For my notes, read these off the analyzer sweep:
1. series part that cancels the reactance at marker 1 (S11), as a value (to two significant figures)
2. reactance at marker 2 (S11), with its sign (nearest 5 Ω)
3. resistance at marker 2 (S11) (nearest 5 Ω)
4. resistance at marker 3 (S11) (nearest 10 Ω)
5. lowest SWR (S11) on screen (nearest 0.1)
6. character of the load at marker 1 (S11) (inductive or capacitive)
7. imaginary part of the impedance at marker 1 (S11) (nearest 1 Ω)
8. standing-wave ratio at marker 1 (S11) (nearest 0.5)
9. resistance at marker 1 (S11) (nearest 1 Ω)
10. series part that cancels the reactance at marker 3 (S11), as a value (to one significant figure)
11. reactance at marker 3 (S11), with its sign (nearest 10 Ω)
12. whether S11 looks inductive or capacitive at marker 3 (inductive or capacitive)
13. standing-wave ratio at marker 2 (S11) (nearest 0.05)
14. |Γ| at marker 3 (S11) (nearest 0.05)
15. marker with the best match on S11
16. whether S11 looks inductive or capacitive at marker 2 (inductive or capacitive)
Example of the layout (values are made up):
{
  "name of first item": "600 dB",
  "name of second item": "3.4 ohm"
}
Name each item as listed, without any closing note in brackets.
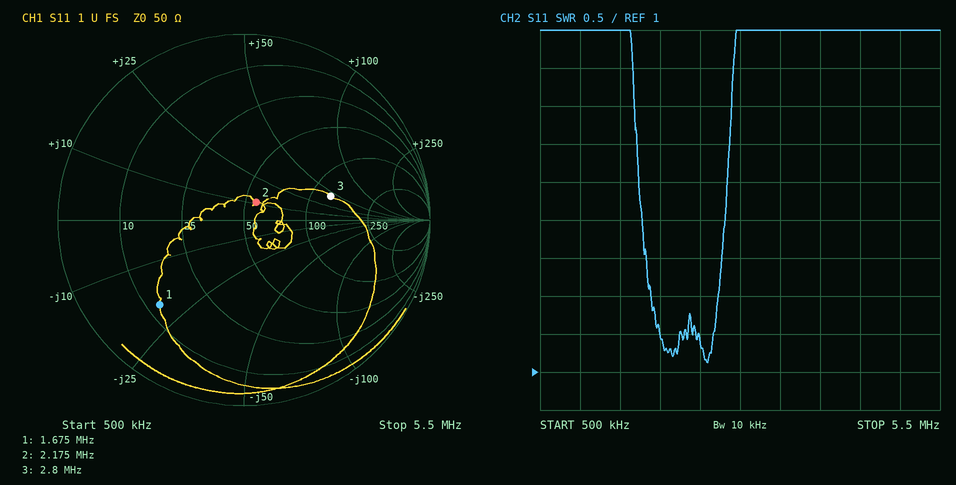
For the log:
{
  "series part that cancels the reactance at marker 1 (S11), as a value": "1.9 µH",
  "reactance at marker 2 (S11), with its sign": "+10 Ω",
  "resistance at marker 2 (S11)": "55 Ω",
  "resistance at marker 3 (S11)": "130 Ω",
  "lowest SWR (S11) on screen": "1.1",
  "character of the load at marker 1 (S11)": "capacitive",
  "imaginary part of the impedance at marker 1 (S11)": "-20 Ω",
  "standing-wave ratio at marker 1 (S11)": "4.5",
  "resistance at marker 1 (S11)": "13 Ω",
  "series part that cancels the reactance at marker 3 (S11), as a value": "1 nF",
  "reactance at marker 3 (S11), with its sign": "+40 Ω",
  "whether S11 looks inductive or capacitive at marker 3": "inductive",
  "standing-wave ratio at marker 2 (S11)": "1.25",
  "|Γ| at marker 3 (S11)": "0.50",
  "marker with the best match on S11": "marker 2",
  "whether S11 looks inductive or capacitive at marker 2": "inductive"
}
